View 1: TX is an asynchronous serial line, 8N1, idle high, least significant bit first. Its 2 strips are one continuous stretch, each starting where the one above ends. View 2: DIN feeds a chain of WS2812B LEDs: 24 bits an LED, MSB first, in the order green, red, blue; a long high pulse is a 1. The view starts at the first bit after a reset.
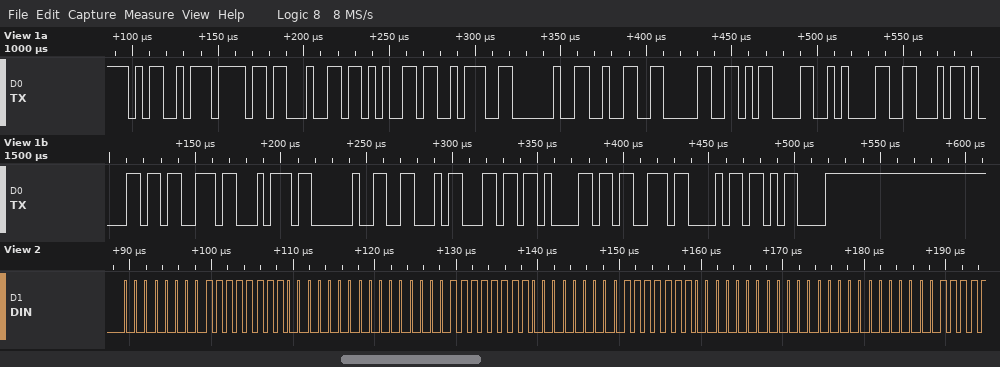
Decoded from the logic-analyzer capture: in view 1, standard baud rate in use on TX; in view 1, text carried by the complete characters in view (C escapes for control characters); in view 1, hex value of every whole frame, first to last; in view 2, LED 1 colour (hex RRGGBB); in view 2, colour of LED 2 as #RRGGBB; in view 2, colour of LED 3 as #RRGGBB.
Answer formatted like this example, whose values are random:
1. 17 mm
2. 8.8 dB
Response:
1. 250000 baud
2. "Mode: 20\r\nFast Flash\r"
3. 4D 6F 64 65 3A 20 32 30 0D 0A 46 61 73 74 20 46 6C 61 73 68 0D
4. #FF0000
5. #FF0000
6. #007F00
